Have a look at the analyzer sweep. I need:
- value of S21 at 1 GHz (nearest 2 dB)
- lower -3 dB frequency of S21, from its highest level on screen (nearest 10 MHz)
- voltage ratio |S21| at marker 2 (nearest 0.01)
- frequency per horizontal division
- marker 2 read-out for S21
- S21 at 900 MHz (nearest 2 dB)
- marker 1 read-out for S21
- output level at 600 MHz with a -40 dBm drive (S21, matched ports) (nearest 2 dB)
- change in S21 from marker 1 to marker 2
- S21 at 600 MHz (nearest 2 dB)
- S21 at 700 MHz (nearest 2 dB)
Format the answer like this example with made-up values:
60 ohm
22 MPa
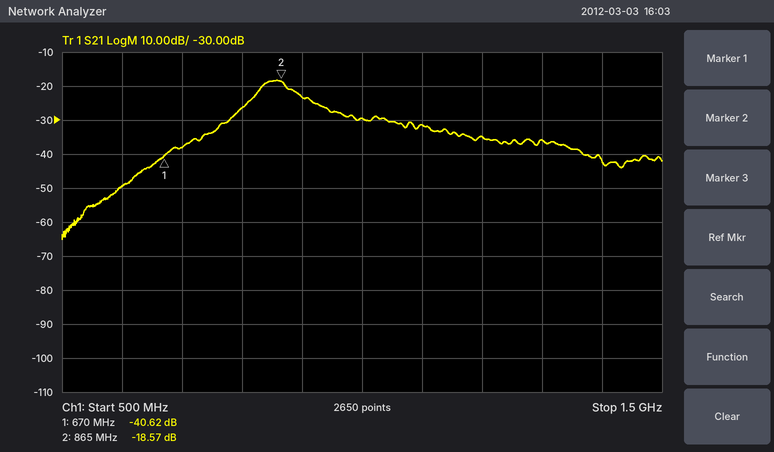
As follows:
-30 dB
830 MHz
0.12
100 MHz
-18.57 dB
-24 dB
-40.62 dB
-90 dBm
22.05 dB
-50 dB
-38 dB
